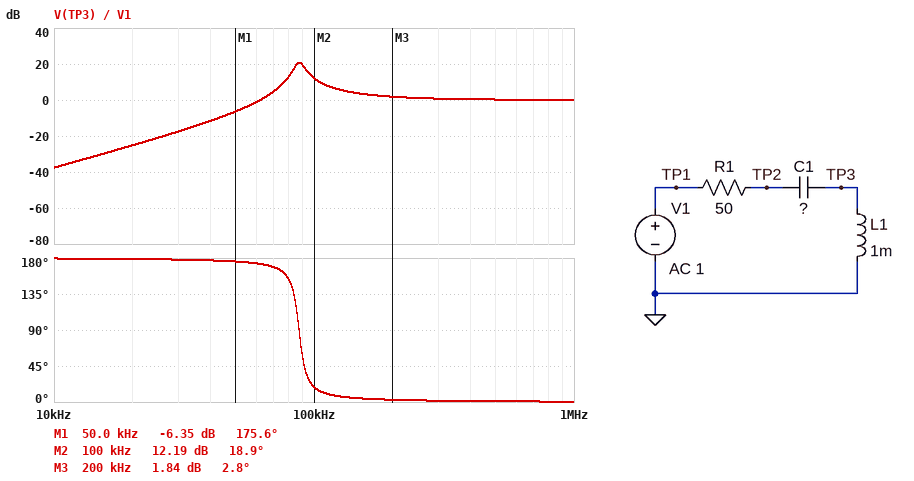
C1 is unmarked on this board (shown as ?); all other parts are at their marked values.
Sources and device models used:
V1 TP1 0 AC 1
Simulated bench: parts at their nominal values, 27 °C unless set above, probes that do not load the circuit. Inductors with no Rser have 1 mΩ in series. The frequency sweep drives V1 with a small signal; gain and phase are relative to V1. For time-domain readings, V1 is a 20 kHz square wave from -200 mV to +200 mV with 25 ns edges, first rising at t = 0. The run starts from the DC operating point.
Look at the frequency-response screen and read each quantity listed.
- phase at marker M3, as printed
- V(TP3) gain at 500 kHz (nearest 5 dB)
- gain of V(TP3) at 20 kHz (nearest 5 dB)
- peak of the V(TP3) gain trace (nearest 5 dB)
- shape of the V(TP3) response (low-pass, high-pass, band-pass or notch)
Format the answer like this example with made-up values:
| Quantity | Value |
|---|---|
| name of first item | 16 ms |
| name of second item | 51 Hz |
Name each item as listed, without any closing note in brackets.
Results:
| Quantity | Value |
|---|---|
| phase at marker M3, as printed | 2.8 deg |
| V(TP3) gain at 500 kHz | 0 dB |
| gain of V(TP3) at 20 kHz | -25 dB |
| peak of the V(TP3) gain trace | 20 dB |
| shape of the V(TP3) response | high-pass |
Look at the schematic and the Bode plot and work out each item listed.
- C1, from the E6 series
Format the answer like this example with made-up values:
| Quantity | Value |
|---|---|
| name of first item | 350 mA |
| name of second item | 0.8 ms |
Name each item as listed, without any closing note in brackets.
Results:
| Quantity | Value |
|---|---|
| C1, from the E6 series | 3.3 nF |
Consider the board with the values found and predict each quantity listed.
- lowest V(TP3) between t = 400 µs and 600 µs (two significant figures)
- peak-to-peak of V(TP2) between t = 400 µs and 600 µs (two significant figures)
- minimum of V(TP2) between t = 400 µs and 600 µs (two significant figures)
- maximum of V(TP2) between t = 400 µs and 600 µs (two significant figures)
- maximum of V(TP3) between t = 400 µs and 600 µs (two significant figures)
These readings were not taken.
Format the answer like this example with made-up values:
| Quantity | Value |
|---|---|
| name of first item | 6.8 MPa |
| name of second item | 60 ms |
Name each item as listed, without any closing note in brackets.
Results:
| Quantity | Value |
|---|---|
| lowest V(TP3) between t = 400 µs and 600 µs | -300 mV |
| peak-to-peak of V(TP2) between t = 400 µs and 600 µs | 440 mV |
| minimum of V(TP2) between t = 400 µs and 600 µs | -220 mV |
| maximum of V(TP2) between t = 400 µs and 600 µs | 220 mV |
| maximum of V(TP3) between t = 400 µs and 600 µs | 300 mV |
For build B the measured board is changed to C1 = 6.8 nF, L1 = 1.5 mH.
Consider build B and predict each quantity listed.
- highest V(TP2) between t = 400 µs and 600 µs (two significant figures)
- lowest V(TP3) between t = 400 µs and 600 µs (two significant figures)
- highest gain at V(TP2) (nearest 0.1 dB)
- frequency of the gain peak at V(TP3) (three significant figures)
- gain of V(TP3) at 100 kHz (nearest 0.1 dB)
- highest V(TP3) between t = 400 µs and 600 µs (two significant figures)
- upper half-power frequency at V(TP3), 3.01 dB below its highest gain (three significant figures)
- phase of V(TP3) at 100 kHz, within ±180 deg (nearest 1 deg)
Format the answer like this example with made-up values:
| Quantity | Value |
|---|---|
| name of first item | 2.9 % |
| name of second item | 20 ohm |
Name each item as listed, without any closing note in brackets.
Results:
| Quantity | Value |
|---|---|
| highest V(TP2) between t = 400 µs and 600 µs | 230 mV |
| lowest V(TP3) between t = 400 µs and 600 µs | -320 mV |
| highest gain at V(TP2) | 0 dB |
| frequency of the gain peak at V(TP3) | 50.0 kHz |
| gain of V(TP3) at 100 kHz | 2.5 dB |
| highest V(TP3) between t = 400 µs and 600 µs | 320 mV |
| upper half-power frequency at V(TP3), 3.01 dB below its highest gain | 52.9 kHz |
| phase of V(TP3) at 100 kHz, within ±180 deg | 4 deg |
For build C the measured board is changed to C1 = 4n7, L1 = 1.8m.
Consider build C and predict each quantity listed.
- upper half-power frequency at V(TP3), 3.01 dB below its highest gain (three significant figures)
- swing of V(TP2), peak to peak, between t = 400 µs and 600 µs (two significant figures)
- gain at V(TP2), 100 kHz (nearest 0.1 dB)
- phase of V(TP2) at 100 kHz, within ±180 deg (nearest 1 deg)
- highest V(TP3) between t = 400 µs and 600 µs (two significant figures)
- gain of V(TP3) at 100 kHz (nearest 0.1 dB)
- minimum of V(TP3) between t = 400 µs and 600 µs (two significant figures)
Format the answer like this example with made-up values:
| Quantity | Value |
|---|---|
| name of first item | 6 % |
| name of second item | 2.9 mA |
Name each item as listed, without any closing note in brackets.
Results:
| Quantity | Value |
|---|---|
| upper half-power frequency at V(TP3), 3.01 dB below its highest gain | 57.2 kHz |
| swing of V(TP2), peak to peak, between t = 400 µs and 600 µs | 470 mV |
| gain at V(TP2), 100 kHz | 0 dB |
| phase of V(TP2) at 100 kHz, within ±180 deg | 4 deg |
| highest V(TP3) between t = 400 µs and 600 µs | 520 mV |
| gain of V(TP3) at 100 kHz | 3.1 dB |
| minimum of V(TP3) between t = 400 µs and 600 µs | -520 mV |
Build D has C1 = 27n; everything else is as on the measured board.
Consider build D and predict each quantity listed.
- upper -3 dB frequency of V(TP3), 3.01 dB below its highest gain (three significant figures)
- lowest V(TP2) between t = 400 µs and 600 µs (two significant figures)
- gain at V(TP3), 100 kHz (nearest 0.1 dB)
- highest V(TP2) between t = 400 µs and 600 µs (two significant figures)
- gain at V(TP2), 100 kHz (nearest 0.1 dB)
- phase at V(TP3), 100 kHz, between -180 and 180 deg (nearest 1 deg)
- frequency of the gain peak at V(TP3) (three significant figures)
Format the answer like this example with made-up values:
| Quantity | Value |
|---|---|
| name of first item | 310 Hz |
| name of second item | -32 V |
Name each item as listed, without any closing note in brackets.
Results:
| Quantity | Value |
|---|---|
| upper -3 dB frequency of V(TP3), 3.01 dB below its highest gain | 36.4 kHz |
| lowest V(TP2) between t = 400 µs and 600 µs | -250 mV |
| gain at V(TP3), 100 kHz | 0.8 dB |
| highest V(TP2) between t = 400 µs and 600 µs | 250 mV |
| gain at V(TP2), 100 kHz | 0 dB |
| phase at V(TP3), 100 kHz, between -180 and 180 deg | 5 deg |
| frequency of the gain peak at V(TP3) | 31.2 kHz |
